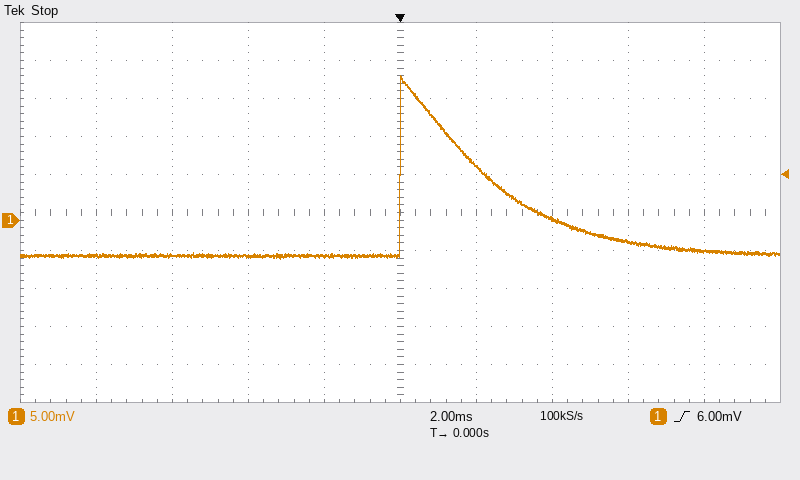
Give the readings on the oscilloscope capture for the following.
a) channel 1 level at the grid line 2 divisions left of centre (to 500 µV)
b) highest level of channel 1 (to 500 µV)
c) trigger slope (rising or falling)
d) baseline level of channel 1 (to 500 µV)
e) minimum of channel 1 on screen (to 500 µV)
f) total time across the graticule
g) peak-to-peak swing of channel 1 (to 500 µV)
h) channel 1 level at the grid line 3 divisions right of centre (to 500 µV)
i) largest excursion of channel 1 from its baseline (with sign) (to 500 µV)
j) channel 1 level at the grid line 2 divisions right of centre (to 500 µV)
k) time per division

-4.5 mV
19.0 mV
rising
-4.5 mV
-5.0 mV
20 ms
24.0 mV
-3.0 mV
+23.5 mV
0.0 mV
2 ms
